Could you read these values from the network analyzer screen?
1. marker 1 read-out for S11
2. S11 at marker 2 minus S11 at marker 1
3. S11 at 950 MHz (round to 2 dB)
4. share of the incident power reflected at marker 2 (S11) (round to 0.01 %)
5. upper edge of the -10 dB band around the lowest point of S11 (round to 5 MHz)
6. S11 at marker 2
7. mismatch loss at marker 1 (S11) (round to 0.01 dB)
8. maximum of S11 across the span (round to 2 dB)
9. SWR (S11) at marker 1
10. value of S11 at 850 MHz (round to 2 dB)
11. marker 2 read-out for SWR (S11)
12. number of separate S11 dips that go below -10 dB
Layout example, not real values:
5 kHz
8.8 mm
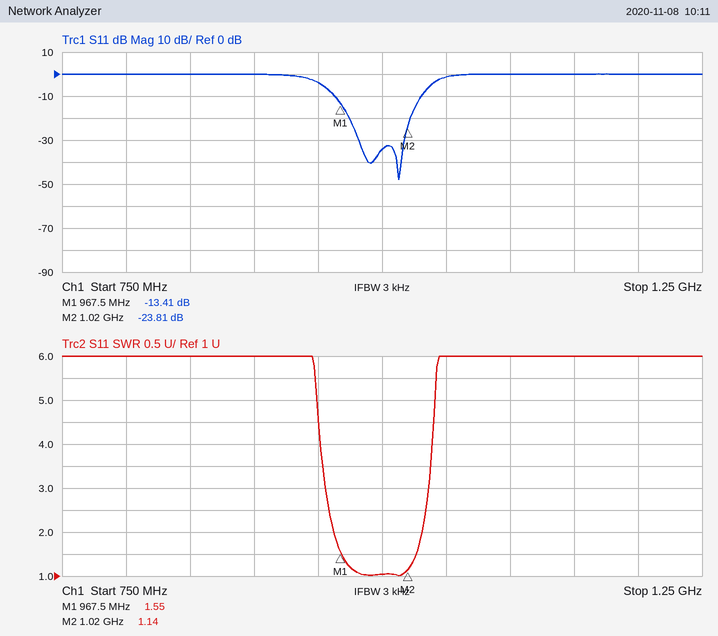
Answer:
-13.41 dB
-10.40 dB
-4 dB
0.42 %
1.030 GHz
-23.81 dB
0.20 dB
0 dB
1.55
0 dB
1.14
2
